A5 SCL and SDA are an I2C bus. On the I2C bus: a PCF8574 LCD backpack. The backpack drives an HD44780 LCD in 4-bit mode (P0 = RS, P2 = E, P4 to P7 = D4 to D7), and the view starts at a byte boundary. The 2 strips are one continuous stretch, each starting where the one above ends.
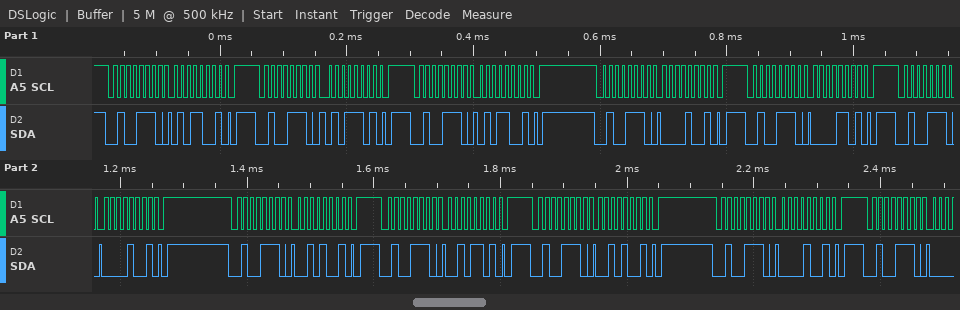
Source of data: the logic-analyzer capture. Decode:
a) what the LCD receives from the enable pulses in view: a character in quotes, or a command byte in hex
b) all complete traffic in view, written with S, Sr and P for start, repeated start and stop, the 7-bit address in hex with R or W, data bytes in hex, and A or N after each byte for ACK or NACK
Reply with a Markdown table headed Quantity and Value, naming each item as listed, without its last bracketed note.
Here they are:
| Quantity | Value |
|---|---|
| what the LCD receives from the enable pulses in view: a character in quotes, or a command byte in hex | 'P' |
| all complete traffic in view, written with S, Sr and P for start, repeated start and stop, the 7-bit address in hex with R or W, data bytes in hex, and A or N after each byte for ACK or NACK | S 27W A 59 A P S 27W A 5D A P S 27W A 59 A P S 27W A 09 A P S 27W A 0D A P S 27W A 09 A P S 27W A 29 A P S 27W A 2D A P S 27W A 29 A P S 27W A 09 A P S 27W A |
